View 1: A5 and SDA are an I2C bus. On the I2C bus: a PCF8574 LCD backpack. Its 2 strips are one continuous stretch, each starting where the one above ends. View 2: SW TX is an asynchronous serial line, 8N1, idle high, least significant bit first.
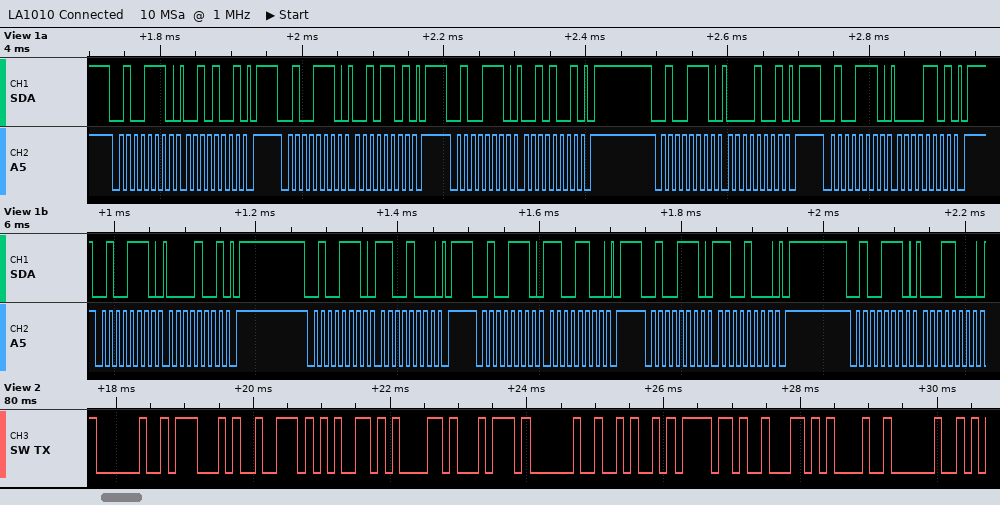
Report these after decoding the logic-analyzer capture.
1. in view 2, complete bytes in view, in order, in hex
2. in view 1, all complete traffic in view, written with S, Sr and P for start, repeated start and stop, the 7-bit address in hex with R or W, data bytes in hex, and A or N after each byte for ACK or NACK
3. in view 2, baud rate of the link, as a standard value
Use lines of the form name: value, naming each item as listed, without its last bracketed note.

in view 2, complete bytes in view, in order, in hex: 20 47 72 65 61 74 20 4A 6F 62 21 20
in view 1, all complete traffic in view, written with S, Sr and P for start, repeated start and stop, the 7-bit address in hex with R or W, data bytes in hex, and A or N after each byte for ACK or NACK: S 27W A 29 A P S 27W A 2D A P S 27W A 29 A P S 27W A 09 A P S 27W A 0D A P S 27W A 09 A P S 27W A C8 A P S 27W A CC A P S 27W A C8 A P S 27W A 18 A
in view 2, baud rate of the link, as a standard value: 9600 baud
